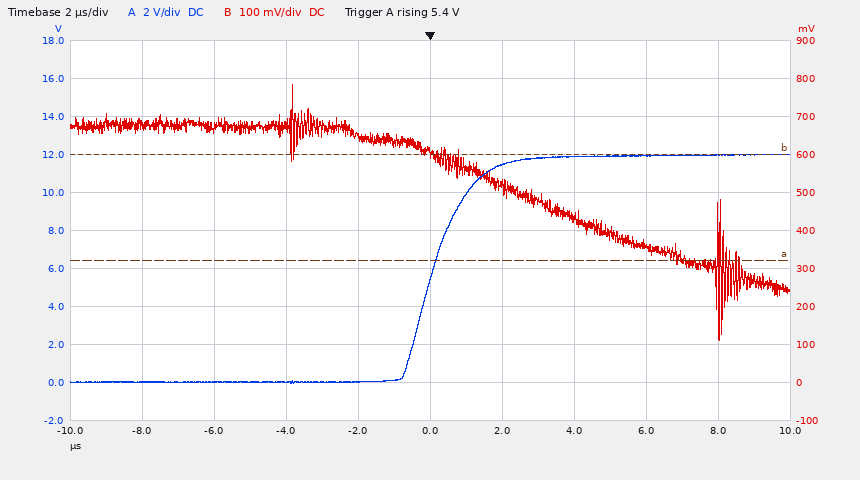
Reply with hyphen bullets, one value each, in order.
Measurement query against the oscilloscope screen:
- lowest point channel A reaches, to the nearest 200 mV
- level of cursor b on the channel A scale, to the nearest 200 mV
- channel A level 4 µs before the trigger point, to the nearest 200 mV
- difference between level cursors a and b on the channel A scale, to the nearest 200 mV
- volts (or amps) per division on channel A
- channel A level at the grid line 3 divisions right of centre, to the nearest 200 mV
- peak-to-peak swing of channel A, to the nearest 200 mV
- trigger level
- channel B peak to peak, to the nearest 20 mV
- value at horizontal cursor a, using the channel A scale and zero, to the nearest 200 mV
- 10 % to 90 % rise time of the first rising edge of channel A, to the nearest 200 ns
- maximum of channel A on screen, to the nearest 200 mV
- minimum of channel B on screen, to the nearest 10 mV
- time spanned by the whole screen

- 0.0 V
- 12.0 V
- 0.0 V
- 5.6 V
- 2 V
- 12.0 V
- 12.0 V
- 5.4 V
- 680 mV
- 6.4 V
- 2.0 µs
- 12.0 V
- 110 mV
- 20 µs
